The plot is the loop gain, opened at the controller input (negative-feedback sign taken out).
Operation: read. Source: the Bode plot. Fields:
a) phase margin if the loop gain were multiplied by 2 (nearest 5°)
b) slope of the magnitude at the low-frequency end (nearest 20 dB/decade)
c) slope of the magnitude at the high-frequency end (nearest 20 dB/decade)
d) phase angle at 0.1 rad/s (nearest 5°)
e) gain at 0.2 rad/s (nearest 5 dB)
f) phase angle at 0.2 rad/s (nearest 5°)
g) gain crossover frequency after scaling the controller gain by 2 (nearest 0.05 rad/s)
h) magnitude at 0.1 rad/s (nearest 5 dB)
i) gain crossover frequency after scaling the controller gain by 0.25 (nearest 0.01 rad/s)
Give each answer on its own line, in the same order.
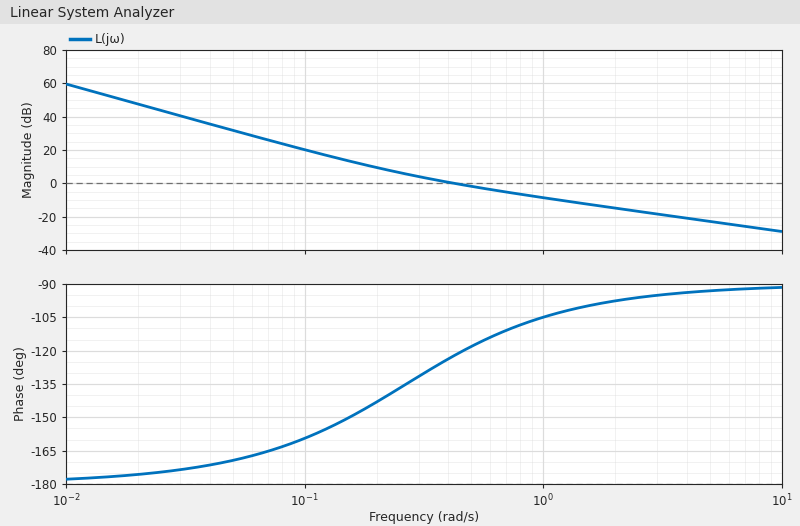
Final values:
70°
-40 dB/decade
-20 dB/decade
-160°
10 dB
-145°
0.75 rad/s
20 dB
0.17 rad/s
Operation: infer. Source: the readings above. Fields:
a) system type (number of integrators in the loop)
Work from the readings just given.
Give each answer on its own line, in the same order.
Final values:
2
